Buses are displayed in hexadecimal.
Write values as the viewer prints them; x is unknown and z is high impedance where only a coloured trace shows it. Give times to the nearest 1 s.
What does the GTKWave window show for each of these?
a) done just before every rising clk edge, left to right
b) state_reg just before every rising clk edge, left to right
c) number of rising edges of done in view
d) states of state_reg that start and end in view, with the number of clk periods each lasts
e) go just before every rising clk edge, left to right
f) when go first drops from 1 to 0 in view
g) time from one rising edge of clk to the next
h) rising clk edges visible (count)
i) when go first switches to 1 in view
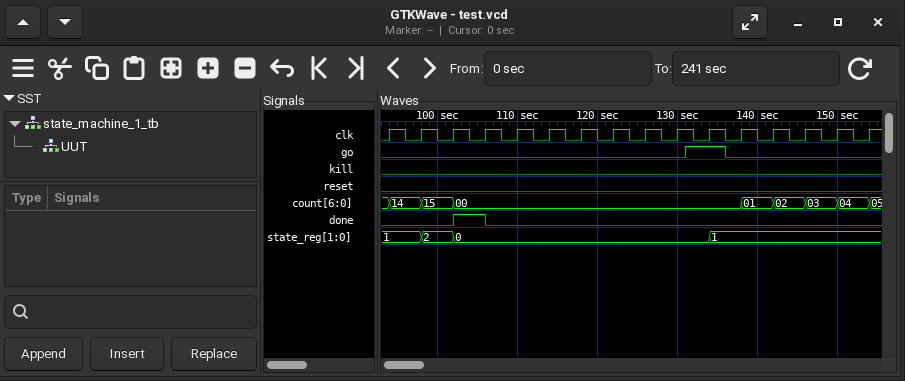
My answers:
0 0 0 1 0 0 0 0 0 0 0 0 0 0 0 0
1, 1, 2, 0, 0, 0, 0, 0, 0, 0, 0, 1, 1, 1, 1, 1
1
2: 1, 0: 8
0 0 0 0 0 0 0 0 0 0 1 0 0 0 0 0
136 s
4 s
16
131 s
